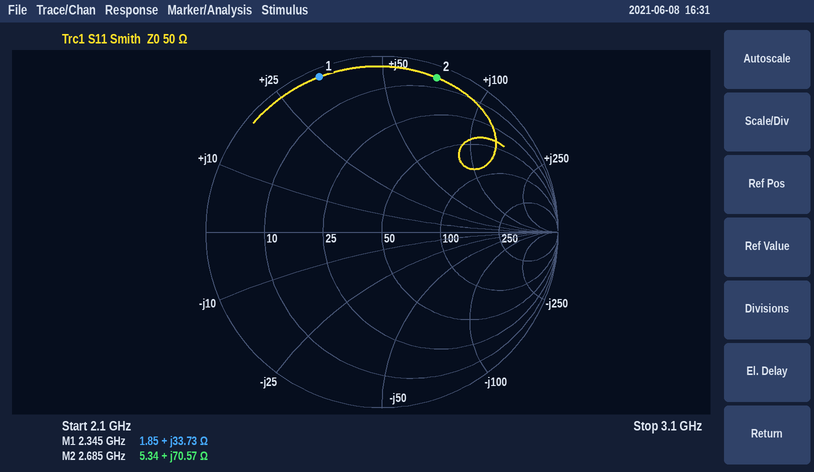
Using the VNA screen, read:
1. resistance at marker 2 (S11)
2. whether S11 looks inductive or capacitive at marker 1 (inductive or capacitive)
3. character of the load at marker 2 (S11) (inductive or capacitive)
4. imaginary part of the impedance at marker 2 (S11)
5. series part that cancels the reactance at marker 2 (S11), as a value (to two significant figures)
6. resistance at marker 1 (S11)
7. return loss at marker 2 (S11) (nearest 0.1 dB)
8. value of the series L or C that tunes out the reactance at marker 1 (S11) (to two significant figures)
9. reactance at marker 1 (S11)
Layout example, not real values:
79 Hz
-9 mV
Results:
5.34 Ω
inductive
inductive
+70.57 Ω
840 fF
1.85 Ω
0.6 dB
2.0 pF
+33.73 Ω
